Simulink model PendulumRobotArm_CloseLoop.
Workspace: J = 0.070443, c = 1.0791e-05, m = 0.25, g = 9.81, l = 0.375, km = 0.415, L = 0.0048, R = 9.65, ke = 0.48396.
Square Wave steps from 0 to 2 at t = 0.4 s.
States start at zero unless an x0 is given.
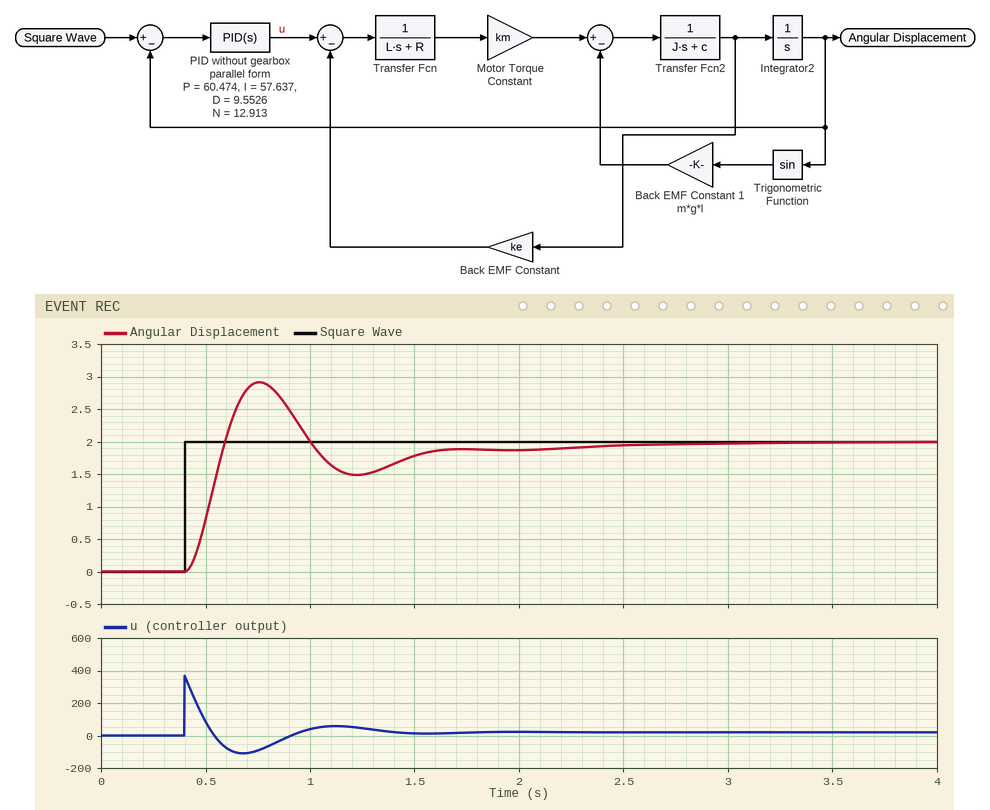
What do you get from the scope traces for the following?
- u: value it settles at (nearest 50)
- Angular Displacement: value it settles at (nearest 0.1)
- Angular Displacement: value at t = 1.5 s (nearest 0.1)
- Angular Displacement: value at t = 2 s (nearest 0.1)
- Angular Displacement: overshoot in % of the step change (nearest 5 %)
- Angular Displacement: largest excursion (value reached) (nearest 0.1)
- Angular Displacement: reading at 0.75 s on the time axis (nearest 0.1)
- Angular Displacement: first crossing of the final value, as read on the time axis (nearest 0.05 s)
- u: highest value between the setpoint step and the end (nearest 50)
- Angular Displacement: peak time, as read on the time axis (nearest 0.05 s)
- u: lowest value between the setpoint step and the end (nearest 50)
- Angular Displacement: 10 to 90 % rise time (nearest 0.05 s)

0
2.0
1.8
1.9
45 %
2.9
2.9
0.60 s
350
0.75 s
-100
0.15 s
